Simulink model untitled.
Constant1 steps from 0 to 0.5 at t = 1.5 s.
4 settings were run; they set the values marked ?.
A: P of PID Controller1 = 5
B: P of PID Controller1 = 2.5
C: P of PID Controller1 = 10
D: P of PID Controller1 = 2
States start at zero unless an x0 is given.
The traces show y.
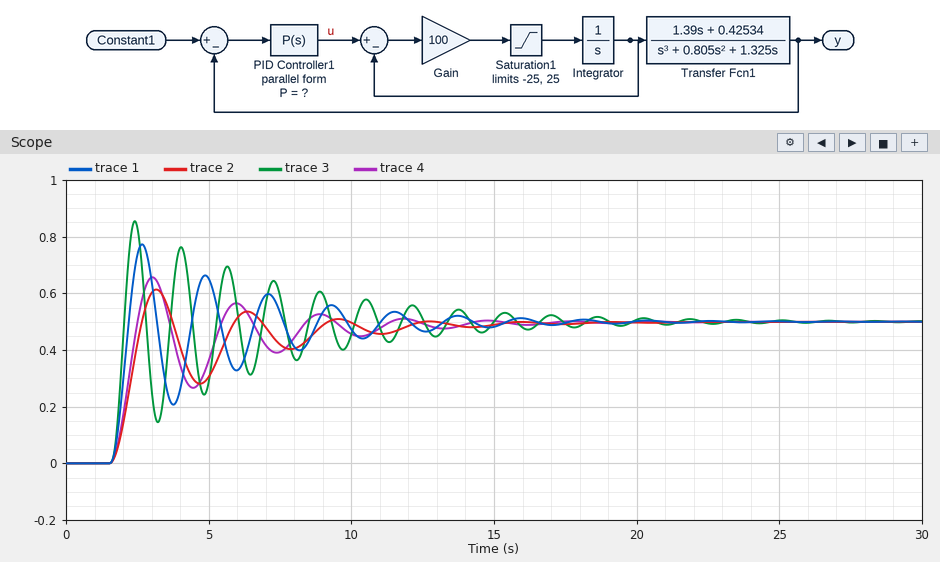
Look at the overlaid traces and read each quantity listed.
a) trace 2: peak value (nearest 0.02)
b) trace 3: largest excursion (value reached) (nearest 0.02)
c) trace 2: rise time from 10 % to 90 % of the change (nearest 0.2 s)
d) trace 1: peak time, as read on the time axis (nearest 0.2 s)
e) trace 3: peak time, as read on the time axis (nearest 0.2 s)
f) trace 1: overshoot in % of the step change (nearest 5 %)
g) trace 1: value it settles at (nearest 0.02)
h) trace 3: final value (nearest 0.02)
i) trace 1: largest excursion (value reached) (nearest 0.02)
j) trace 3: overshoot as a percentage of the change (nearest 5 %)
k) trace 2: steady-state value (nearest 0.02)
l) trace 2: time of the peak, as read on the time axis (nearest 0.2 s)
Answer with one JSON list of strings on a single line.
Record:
["0.62", "0.86", "0.8 s", "2.6 s", "2.4 s", "55 %", "0.50", "0.50", "0.78", "70 %", "0.50", "3.2 s"]
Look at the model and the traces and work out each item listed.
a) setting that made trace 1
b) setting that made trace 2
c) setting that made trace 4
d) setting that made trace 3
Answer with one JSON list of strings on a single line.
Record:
["A", "D", "B", "C"]
